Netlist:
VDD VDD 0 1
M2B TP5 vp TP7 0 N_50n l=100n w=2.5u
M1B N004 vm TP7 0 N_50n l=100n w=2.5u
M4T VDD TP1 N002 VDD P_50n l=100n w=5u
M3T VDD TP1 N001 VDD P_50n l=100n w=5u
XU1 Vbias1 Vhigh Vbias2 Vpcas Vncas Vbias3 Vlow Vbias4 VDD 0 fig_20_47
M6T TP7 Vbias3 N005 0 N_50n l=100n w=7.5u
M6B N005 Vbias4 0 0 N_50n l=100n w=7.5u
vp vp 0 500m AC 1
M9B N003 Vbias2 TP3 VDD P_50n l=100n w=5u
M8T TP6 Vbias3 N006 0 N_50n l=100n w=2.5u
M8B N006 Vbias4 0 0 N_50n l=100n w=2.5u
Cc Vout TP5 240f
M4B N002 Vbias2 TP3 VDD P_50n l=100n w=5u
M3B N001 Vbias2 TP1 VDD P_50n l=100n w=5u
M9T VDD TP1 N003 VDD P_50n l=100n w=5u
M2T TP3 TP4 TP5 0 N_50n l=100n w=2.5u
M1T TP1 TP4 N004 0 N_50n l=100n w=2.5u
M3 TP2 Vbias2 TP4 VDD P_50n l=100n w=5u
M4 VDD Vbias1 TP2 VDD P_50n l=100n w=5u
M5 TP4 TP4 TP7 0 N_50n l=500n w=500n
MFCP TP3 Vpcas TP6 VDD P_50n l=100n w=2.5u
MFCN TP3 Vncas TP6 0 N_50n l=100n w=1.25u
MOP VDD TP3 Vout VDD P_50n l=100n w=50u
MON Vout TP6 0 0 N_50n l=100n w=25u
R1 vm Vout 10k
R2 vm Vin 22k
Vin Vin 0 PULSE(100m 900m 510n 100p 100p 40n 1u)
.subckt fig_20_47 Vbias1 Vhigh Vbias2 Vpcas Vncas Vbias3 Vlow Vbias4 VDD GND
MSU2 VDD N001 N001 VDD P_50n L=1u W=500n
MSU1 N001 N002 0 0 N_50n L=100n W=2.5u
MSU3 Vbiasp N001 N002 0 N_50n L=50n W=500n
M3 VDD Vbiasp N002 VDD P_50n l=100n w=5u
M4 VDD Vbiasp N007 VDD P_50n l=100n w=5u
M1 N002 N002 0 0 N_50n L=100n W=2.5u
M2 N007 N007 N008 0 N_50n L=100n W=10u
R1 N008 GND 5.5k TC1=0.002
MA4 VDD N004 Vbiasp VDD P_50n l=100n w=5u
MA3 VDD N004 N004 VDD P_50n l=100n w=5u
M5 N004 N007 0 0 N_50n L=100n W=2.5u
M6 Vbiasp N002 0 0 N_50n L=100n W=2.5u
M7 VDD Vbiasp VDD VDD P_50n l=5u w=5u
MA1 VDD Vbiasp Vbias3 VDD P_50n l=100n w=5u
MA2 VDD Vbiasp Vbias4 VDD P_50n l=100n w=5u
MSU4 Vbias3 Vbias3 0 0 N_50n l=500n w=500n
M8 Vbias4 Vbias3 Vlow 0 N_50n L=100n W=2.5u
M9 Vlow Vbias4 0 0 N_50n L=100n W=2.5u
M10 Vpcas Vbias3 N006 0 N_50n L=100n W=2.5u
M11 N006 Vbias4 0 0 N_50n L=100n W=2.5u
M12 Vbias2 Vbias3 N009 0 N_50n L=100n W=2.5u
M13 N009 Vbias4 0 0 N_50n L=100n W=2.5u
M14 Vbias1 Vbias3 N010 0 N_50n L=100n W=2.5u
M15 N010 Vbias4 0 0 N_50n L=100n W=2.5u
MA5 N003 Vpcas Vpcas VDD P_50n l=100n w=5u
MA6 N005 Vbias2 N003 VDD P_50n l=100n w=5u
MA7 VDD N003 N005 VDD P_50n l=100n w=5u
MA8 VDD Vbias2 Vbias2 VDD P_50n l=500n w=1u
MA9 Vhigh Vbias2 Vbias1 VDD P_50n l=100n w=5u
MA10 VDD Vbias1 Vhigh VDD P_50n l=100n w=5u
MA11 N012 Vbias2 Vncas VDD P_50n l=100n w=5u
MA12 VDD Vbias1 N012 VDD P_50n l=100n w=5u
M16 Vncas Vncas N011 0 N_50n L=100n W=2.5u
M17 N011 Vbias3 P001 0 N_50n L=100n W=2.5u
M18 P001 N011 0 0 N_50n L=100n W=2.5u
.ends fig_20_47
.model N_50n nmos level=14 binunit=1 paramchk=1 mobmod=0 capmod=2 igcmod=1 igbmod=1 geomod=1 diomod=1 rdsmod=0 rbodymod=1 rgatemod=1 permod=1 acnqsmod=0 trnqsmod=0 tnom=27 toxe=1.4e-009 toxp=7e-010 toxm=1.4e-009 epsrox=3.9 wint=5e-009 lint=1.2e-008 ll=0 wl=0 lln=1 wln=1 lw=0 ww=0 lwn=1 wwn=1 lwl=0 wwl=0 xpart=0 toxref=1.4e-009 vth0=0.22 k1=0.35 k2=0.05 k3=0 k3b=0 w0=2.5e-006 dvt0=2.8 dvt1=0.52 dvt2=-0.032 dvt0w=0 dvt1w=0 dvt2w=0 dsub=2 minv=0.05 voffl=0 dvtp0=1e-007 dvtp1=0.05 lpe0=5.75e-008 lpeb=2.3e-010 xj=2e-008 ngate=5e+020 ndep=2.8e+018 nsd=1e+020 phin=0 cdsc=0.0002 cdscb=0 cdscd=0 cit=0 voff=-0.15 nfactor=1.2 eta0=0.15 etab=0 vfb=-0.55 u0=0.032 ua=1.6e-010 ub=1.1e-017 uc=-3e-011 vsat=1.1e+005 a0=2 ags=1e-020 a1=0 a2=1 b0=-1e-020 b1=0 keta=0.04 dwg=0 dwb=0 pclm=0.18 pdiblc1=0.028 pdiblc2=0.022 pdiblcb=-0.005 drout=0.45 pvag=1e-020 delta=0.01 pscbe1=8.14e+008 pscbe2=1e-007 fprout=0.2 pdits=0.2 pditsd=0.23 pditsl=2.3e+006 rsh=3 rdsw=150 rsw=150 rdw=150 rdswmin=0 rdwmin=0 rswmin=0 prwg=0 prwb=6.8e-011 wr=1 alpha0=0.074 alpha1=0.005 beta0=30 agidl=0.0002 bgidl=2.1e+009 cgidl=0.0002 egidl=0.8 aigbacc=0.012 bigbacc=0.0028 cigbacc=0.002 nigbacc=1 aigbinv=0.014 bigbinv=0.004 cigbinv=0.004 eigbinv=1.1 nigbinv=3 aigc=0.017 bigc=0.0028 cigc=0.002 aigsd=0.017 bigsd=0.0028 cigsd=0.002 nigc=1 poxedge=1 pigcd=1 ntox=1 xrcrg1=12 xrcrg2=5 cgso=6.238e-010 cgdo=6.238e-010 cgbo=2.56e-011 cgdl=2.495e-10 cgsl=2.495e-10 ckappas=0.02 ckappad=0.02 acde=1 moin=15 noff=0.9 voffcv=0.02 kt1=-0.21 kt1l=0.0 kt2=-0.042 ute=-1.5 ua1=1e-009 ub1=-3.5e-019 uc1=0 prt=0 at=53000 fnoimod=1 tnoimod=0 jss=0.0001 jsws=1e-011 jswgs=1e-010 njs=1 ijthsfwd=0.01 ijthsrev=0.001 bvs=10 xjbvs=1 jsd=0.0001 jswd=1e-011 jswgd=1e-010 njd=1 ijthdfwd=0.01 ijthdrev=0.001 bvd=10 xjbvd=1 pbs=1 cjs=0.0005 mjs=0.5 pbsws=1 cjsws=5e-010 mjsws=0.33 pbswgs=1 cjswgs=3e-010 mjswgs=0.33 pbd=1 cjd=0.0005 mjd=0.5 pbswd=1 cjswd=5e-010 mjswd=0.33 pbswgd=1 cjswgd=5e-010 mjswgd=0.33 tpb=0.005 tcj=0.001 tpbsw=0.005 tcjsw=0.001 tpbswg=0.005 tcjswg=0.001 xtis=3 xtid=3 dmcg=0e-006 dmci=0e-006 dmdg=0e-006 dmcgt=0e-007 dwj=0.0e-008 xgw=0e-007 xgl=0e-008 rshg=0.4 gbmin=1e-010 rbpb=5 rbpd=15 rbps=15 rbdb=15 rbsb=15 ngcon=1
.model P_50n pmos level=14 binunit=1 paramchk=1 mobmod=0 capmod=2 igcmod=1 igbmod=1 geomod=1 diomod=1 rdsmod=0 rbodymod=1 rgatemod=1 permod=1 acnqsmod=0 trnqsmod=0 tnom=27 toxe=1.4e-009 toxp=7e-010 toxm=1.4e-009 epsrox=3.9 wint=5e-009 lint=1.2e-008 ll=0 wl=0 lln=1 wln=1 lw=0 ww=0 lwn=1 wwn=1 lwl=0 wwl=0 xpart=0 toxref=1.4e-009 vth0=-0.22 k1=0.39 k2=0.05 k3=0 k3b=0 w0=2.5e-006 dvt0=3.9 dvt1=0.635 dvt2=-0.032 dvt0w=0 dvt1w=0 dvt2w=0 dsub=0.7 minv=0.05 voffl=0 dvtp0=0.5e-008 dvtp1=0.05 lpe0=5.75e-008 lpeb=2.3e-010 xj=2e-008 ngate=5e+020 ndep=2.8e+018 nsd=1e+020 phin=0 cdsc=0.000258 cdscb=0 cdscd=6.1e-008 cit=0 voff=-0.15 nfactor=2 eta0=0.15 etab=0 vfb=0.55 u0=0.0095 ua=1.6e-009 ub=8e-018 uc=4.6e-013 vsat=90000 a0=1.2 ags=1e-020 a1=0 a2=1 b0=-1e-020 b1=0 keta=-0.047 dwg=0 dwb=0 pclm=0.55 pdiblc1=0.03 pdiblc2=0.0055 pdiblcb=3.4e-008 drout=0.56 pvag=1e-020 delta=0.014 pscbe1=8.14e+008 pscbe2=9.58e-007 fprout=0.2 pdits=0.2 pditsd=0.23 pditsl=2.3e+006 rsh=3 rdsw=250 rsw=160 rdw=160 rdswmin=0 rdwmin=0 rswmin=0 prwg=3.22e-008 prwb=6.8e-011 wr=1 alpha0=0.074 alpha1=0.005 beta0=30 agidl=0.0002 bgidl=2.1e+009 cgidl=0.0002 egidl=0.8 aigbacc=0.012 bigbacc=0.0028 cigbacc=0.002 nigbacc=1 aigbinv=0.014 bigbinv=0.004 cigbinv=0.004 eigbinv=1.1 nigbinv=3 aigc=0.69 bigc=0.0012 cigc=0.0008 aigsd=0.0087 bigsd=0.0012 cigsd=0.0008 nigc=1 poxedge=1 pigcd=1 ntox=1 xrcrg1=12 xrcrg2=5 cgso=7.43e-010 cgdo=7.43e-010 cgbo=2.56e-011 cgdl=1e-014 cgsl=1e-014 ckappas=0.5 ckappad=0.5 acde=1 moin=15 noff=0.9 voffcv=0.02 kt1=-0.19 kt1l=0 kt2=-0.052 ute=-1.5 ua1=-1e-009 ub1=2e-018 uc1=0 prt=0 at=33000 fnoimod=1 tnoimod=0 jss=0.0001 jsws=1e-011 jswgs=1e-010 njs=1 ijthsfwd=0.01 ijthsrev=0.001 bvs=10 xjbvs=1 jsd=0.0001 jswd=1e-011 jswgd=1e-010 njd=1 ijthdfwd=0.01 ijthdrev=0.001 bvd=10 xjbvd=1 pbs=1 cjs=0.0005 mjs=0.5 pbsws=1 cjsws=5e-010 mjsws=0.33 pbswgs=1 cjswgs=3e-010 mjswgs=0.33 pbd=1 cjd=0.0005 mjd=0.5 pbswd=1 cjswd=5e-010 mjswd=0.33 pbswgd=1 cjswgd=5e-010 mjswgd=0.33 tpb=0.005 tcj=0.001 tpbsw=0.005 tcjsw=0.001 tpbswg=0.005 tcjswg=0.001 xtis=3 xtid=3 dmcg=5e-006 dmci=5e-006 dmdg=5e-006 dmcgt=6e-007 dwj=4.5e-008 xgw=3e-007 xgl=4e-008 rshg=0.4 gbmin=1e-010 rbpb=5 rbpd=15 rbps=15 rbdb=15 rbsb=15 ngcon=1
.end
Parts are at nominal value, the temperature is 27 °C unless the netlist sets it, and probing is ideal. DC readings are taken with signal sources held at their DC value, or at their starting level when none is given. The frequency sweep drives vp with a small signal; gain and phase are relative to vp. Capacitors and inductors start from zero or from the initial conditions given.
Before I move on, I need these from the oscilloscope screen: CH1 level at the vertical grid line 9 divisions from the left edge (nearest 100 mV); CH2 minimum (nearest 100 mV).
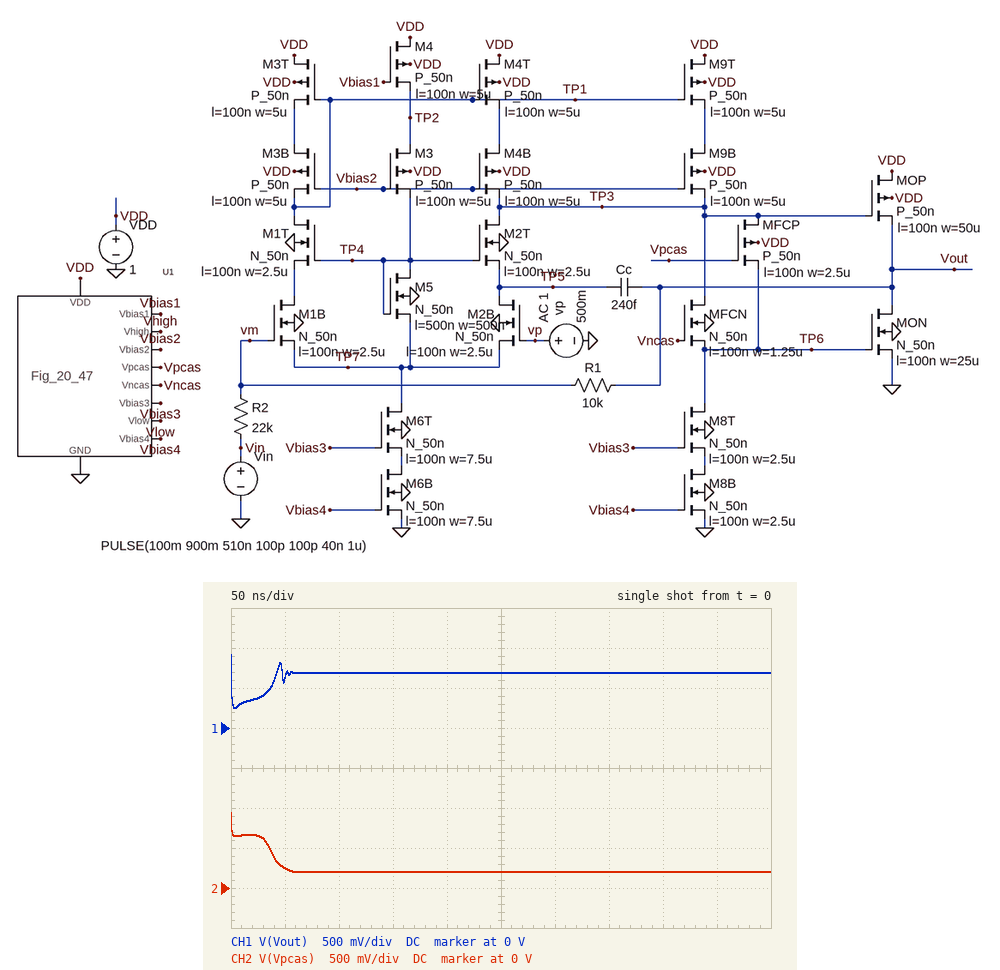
700 mV
200 mV
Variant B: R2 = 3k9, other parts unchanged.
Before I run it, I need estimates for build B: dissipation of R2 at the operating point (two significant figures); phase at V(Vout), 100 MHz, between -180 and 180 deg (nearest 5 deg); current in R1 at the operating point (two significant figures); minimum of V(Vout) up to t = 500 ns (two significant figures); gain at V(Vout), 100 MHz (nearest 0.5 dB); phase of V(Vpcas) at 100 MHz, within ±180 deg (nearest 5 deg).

16 µW
-160 deg
64 µA
230 mV
-69.0 dB
-80 deg
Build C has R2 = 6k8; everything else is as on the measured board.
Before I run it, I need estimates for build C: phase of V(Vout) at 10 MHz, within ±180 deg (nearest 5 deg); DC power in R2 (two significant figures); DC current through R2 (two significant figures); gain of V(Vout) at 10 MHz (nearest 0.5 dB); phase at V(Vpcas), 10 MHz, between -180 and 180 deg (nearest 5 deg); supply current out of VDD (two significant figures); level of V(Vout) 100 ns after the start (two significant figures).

-35 deg
19 µW
53 µA
-53.0 dB
-100 deg
200 µA
1.0 V
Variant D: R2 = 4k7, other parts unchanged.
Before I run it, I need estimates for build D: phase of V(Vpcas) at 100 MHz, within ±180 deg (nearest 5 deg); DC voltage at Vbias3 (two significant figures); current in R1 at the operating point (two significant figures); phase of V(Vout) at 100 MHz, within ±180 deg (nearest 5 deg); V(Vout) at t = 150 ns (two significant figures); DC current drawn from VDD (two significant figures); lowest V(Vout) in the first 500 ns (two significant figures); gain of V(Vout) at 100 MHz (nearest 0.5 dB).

-85 deg
540 mV
61 µA
-145 deg
1.0 V
200 µA
230 mV
-62.0 dB
